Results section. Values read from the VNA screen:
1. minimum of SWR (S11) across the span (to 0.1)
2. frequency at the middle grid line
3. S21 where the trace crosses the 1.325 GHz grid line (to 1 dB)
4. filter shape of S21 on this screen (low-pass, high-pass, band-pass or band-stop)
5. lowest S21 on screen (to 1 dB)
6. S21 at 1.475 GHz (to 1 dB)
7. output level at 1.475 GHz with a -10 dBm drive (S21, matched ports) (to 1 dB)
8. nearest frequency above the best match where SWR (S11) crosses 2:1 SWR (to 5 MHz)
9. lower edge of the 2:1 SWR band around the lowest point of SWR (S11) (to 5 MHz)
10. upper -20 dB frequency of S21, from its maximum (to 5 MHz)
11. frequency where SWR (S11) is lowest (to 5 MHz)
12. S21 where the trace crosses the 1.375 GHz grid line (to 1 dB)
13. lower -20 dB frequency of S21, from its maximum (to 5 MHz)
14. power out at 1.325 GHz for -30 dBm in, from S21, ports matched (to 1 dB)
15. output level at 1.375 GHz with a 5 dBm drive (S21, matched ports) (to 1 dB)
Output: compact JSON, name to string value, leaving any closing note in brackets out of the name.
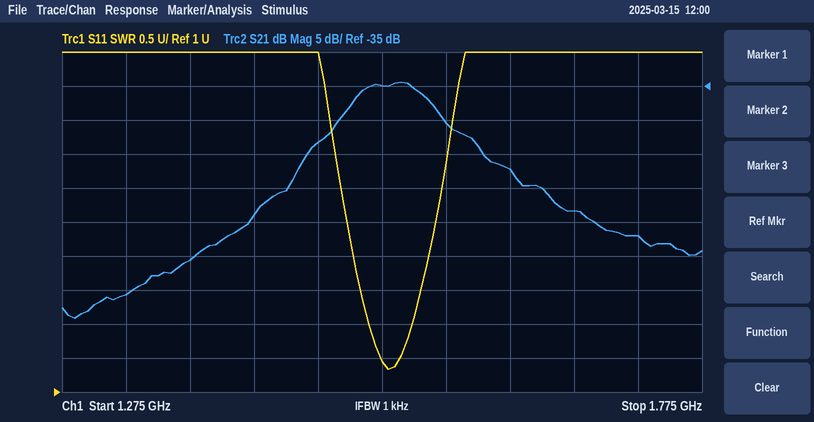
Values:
{"minimum of SWR (S11) across the span": "1.3", "frequency at the middle grid line": "1.525 GHz", "S21 where the trace crosses the 1.325 GHz grid line": "-66 dB", "filter shape of S21 on this screen": "band-pass", "lowest S21 on screen": "-69 dB", "S21 at 1.475 GHz": "-43 dB", "output level at 1.475 GHz with a -10 dBm drive (S21, matched ports)": "-53 dBm", "nearest frequency above the best match where SWR (S11) crosses 2:1 SWR": "1.550 GHz", "lower edge of the 2:1 SWR band around the lowest point of SWR (S11)": "1.515 GHz", "upper -20 dB frequency of S21, from its maximum": "1.685 GHz", "frequency where SWR (S11) is lowest": "1.530 GHz", "S21 where the trace crosses the 1.375 GHz grid line": "-61 dB", "lower -20 dB frequency of S21, from its maximum": "1.425 GHz", "power out at 1.325 GHz for -30 dBm in, from S21, ports matched": "-96 dBm", "output level at 1.375 GHz with a 5 dBm drive (S21, matched ports)": "-56 dBm"}
